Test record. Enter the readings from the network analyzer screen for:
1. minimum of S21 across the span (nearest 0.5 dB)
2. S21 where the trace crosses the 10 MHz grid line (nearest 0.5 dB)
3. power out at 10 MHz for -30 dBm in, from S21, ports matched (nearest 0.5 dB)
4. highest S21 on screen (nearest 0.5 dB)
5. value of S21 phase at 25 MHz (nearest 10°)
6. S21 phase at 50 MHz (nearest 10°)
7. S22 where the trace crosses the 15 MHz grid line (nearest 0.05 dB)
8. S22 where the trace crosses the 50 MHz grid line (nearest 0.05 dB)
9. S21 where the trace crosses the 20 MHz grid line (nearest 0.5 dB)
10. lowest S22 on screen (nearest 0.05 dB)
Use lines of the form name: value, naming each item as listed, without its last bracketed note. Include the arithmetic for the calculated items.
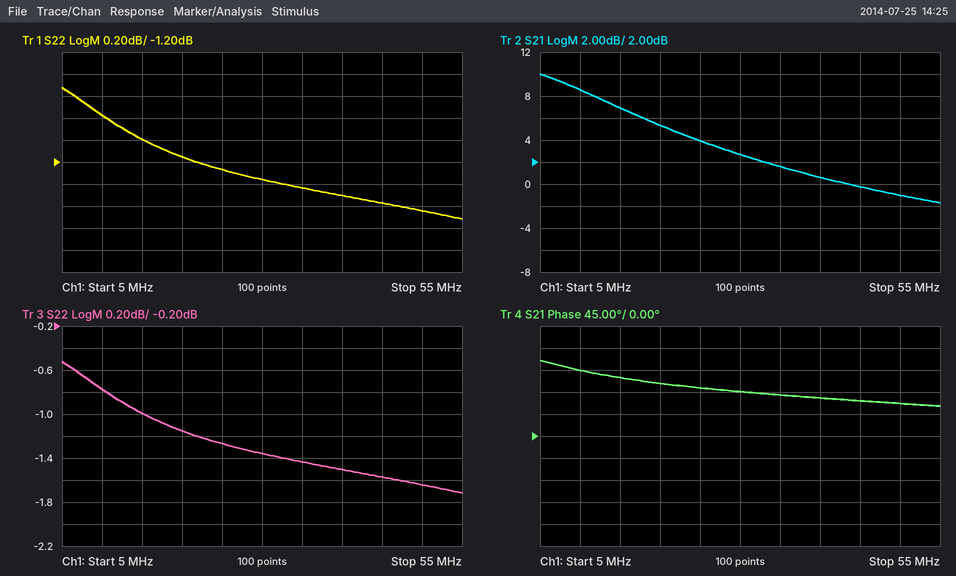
minimum of S21 across the span: -1.5 dB
S21 where the trace crosses the 10 MHz grid line: 8.5 dB
power out at 10 MHz for -30 dBm in, from S21, ports matched: -30 dBm + (8.5 dB) = -21.5 dBm
highest S21 on screen: 10.0 dB
value of S21 phase at 25 MHz: 100°
S21 phase at 50 MHz: 70°
S22 where the trace crosses the 15 MHz grid line: -1.00 dB
S22 where the trace crosses the 50 MHz grid line: -1.65 dB
S21 where the trace crosses the 20 MHz grid line: 5.5 dB
lowest S22 on screen: -1.70 dB
